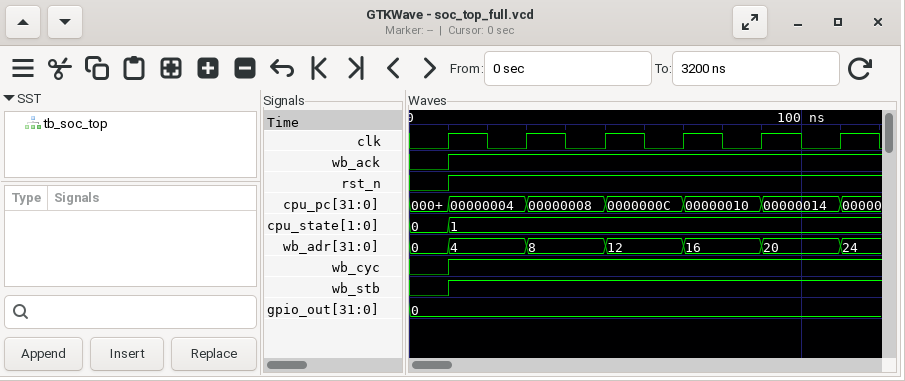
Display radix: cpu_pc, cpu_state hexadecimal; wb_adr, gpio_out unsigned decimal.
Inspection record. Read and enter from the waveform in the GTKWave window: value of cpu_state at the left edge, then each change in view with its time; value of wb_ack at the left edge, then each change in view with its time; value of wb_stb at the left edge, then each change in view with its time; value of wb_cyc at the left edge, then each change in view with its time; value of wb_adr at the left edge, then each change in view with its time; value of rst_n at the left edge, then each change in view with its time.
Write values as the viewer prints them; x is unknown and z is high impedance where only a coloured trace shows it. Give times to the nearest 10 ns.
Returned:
0, 1 at 10 ns
0, 1 at 10 ns
0, 1 at 10 ns
0, 1 at 10 ns
0, 4 at 10 ns, 8 at 30 ns, 12 at 50 ns, 16 at 70 ns, 20 at 90 ns, 24 at 110 ns
0, 1 at 10 ns
